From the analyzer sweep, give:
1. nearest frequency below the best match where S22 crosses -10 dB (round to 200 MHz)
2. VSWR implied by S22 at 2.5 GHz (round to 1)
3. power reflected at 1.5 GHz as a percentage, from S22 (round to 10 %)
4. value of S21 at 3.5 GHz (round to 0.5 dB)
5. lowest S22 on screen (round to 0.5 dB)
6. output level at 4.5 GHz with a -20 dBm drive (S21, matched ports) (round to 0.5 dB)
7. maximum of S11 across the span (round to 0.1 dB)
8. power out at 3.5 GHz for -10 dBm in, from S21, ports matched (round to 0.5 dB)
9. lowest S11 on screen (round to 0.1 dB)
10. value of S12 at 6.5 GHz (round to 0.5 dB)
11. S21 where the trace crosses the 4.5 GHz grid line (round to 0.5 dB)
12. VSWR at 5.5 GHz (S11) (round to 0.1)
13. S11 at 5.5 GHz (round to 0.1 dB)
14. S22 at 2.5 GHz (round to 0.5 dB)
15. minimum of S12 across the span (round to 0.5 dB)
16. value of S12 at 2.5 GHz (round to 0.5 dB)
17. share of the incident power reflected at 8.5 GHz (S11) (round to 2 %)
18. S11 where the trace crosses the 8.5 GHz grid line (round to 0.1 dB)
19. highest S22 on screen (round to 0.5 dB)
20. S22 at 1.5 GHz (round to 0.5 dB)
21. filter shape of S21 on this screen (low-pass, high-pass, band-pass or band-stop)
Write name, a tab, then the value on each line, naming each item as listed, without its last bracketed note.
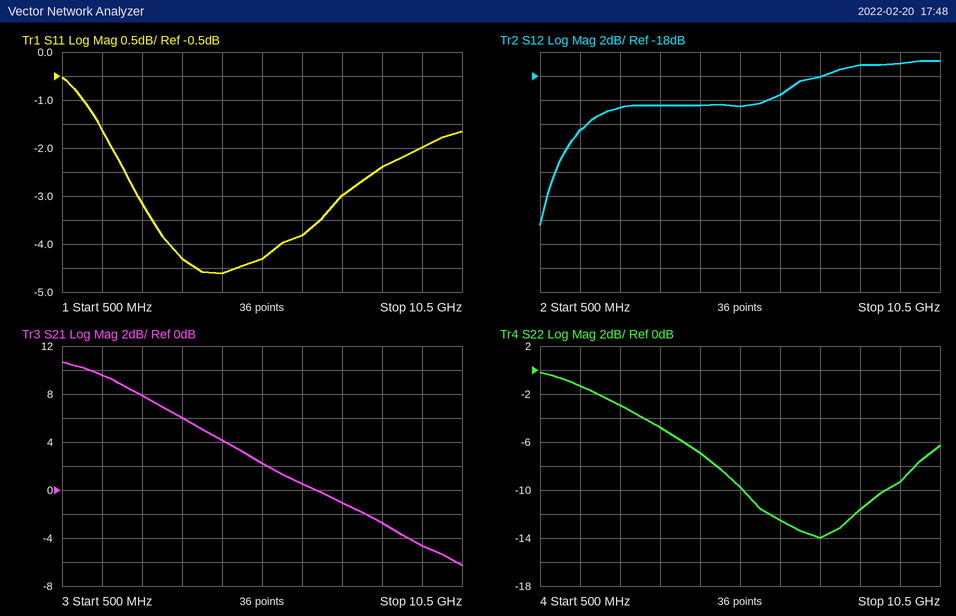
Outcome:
nearest frequency below the best match where S22 crosses -10 dB	5.6 GHz
VSWR implied by S22 at 2.5 GHz	6
power reflected at 1.5 GHz as a percentage, from S22	70 %
value of S21 at 3.5 GHz	6.0 dB
lowest S22 on screen	-14.0 dB
output level at 4.5 GHz with a -20 dBm drive (S21, matched ports)	-16.0 dBm
maximum of S11 across the span	-0.5 dB
power out at 3.5 GHz for -10 dBm in, from S21, ports matched	-4.0 dBm
lowest S11 on screen	-4.6 dB
value of S12 at 6.5 GHz	-19.5 dB
S21 where the trace crosses the 4.5 GHz grid line	4.0 dB
VSWR at 5.5 GHz (S11)	4.1
S11 at 5.5 GHz	-4.3 dB
S22 at 2.5 GHz	-3.0 dB
minimum of S12 across the span	-30.5 dB
value of S12 at 2.5 GHz	-20.5 dB
share of the incident power reflected at 8.5 GHz (S11)	58 %
S11 where the trace crosses the 8.5 GHz grid line	-2.4 dB
highest S22 on screen	0.0 dB
S22 at 1.5 GHz	-1.5 dB
filter shape of S21 on this screen	low-pass
